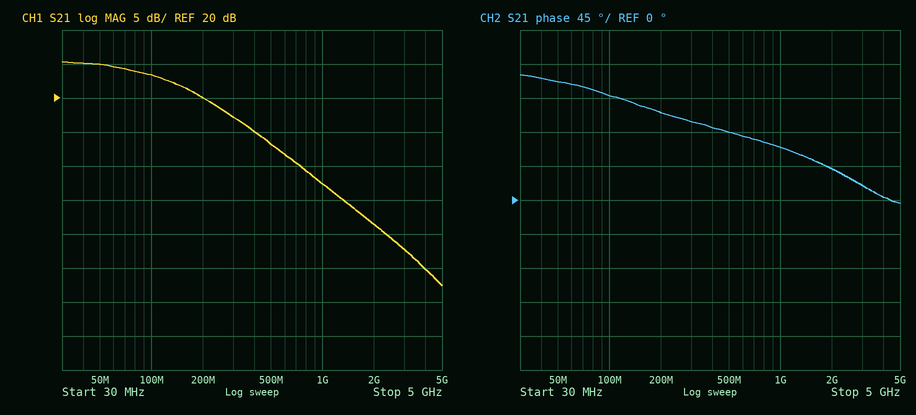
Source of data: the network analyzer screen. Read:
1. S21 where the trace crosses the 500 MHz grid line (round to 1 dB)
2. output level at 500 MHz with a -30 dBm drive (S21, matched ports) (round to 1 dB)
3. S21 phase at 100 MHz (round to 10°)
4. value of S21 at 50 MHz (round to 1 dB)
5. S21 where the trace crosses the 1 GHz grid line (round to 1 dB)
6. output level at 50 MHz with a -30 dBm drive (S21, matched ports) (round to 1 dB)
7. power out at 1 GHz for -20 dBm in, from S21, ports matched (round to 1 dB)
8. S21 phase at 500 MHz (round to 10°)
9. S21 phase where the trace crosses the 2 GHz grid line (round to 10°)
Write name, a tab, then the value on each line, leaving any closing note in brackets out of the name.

S21 where the trace crosses the 500 MHz grid line	13 dB
output level at 500 MHz with a -30 dBm drive (S21, matched ports)	-17 dBm
S21 phase at 100 MHz	140°
value of S21 at 50 MHz	25 dB
S21 where the trace crosses the 1 GHz grid line	7 dB
output level at 50 MHz with a -30 dBm drive (S21, matched ports)	-5 dBm
power out at 1 GHz for -20 dBm in, from S21, ports matched	-13 dBm
S21 phase at 500 MHz	90°
S21 phase where the trace crosses the 2 GHz grid line	40°
